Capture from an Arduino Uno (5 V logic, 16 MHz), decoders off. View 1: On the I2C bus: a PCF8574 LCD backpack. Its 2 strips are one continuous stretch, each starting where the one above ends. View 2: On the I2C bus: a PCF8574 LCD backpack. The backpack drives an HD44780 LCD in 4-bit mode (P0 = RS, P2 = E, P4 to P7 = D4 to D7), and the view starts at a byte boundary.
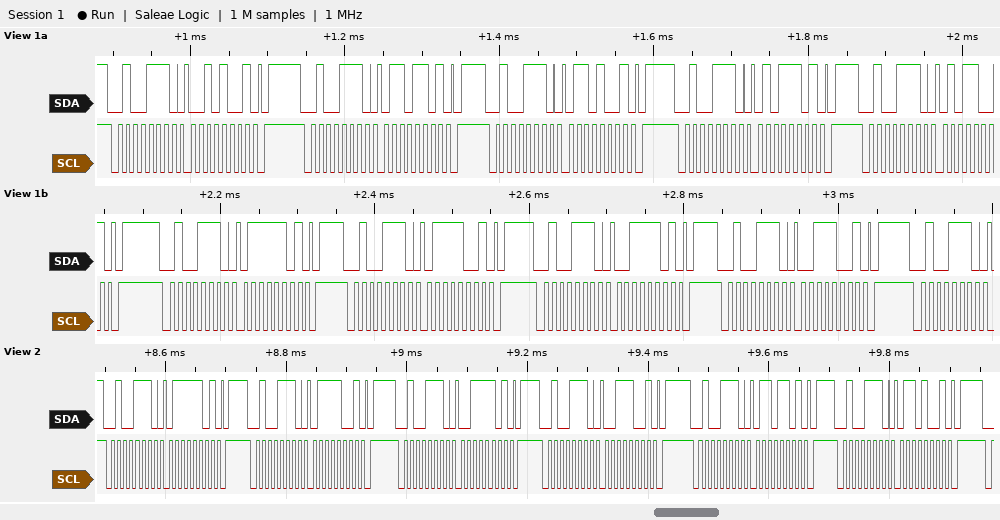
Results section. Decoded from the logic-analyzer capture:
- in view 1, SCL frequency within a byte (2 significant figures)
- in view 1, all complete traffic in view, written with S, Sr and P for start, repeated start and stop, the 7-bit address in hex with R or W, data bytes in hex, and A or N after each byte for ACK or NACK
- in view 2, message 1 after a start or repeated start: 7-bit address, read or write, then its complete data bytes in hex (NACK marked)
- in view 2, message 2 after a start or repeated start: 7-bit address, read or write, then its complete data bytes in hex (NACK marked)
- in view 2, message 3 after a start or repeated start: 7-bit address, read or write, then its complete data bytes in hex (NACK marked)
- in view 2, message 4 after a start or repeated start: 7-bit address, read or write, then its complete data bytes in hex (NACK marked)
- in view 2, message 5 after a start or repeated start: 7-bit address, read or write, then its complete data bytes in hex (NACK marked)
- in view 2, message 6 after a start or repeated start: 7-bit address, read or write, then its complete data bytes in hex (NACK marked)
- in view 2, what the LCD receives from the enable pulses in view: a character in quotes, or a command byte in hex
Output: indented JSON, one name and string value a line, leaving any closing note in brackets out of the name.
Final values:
{
  "in view 1, SCL frequency within a byte": "100 kHz",
  "in view 1, all complete traffic in view, written with S, Sr and P for start, repeated start and stop, the 7-bit address in hex with R or W, data bytes in hex, and A or N after each byte for ACK or NACK": "S 27W A 29 A P S 27W A 6D A P S 27W A 69 A P S 27W A 5D A P S 27W A 59 A P S 27W A 7D A P S 27W A 79 A P S 27W A 3D A P S 27W A 39 A P S 27W A",
  "in view 2, message 1 after a start or repeated start: 7-bit address, read or write, then its complete data bytes in hex": "0x27 write: 7D",
  "in view 2, message 2 after a start or repeated start: 7-bit address, read or write, then its complete data bytes in hex": "0x27 write: 79",
  "in view 2, message 3 after a start or repeated start: 7-bit address, read or write, then its complete data bytes in hex": "0x27 write: 3D",
  "in view 2, message 4 after a start or repeated start: 7-bit address, read or write, then its complete data bytes in hex": "0x27 write: 39",
  "in view 2, message 5 after a start or repeated start: 7-bit address, read or write, then its complete data bytes in hex": "0x27 write: 6D",
  "in view 2, message 6 after a start or repeated start: 7-bit address, read or write, then its complete data bytes in hex": "0x27 write: 69",
  "in view 2, what the LCD receives from the enable pulses in view: a character in quotes, or a command byte in hex": "'s'"
}
